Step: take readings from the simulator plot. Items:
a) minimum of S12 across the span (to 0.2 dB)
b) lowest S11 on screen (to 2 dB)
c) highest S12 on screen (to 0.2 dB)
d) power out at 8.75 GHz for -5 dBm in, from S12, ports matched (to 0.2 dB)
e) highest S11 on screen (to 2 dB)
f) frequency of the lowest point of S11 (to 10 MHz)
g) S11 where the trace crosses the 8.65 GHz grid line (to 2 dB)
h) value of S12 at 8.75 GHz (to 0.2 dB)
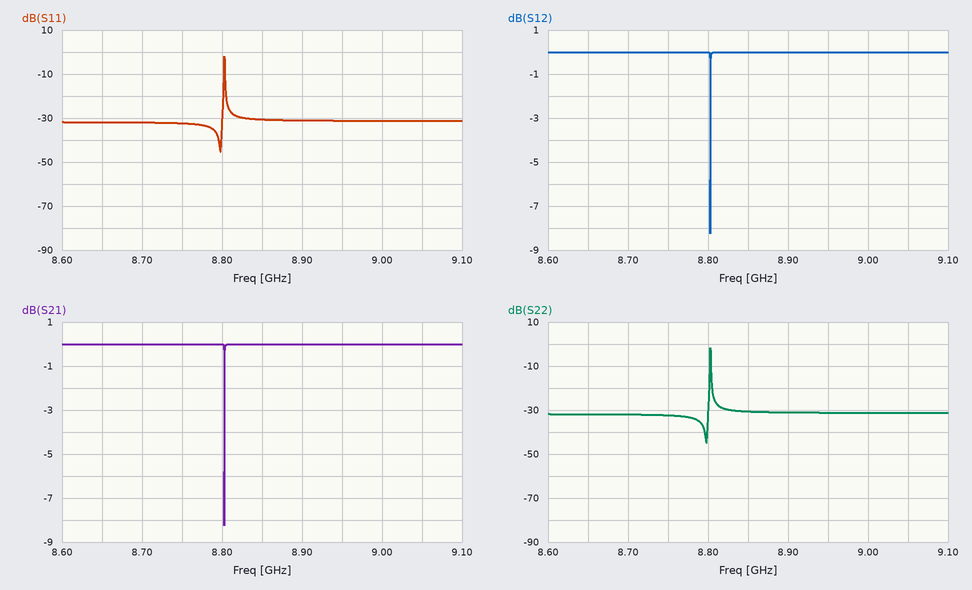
-8.2 dB
-46 dB
0.0 dB
-5.0 dBm
-2 dB
8.80 GHz
-32 dB
0.0 dB
